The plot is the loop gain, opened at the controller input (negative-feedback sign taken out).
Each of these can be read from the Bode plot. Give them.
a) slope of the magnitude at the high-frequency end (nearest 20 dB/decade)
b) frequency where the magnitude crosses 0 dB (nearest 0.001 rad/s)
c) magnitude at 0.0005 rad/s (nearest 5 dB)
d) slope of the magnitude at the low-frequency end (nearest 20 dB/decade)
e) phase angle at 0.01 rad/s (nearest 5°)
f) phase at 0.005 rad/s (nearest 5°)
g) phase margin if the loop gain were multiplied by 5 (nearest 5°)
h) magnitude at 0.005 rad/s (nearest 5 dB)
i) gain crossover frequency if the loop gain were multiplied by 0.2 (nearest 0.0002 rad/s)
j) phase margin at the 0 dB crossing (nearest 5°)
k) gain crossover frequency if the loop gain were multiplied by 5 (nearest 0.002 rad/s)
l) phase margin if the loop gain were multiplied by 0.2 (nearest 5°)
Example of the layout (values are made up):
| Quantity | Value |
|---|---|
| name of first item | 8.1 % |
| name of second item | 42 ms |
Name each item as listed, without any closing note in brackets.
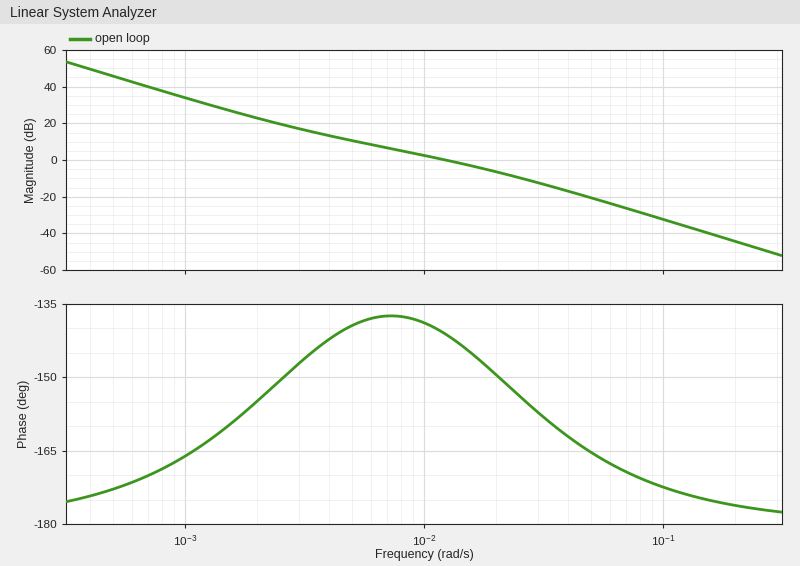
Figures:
| Quantity | Value |
|---|---|
| slope of the magnitude at the high-frequency end | -40 dB/decade |
| frequency where the magnitude crosses 0 dB | 0.012 rad/s |
| magnitude at 0.0005 rad/s | 45 dB |
| slope of the magnitude at the low-frequency end | -40 dB/decade |
| phase angle at 0.01 rad/s | -140° |
| phase at 0.005 rad/s | -140° |
| phase margin if the loop gain were multiplied by 5 | 20° |
| magnitude at 0.005 rad/s | 10 dB |
| gain crossover frequency if the loop gain were multiplied by 0.2 | 0.0038 rad/s |
| phase margin at the 0 dB crossing | 40° |
| gain crossover frequency if the loop gain were multiplied by 5 | 0.034 rad/s |
| phase margin if the loop gain were multiplied by 0.2 | 35° |
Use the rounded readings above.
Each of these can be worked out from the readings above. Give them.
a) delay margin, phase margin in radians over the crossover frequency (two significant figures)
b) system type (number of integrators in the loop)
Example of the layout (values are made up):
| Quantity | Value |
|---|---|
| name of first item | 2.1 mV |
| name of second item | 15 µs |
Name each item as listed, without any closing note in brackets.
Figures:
| Quantity | Value |
|---|---|
| delay margin, phase margin in radians over the crossover frequency | 58 s |
| system type | 2 |
